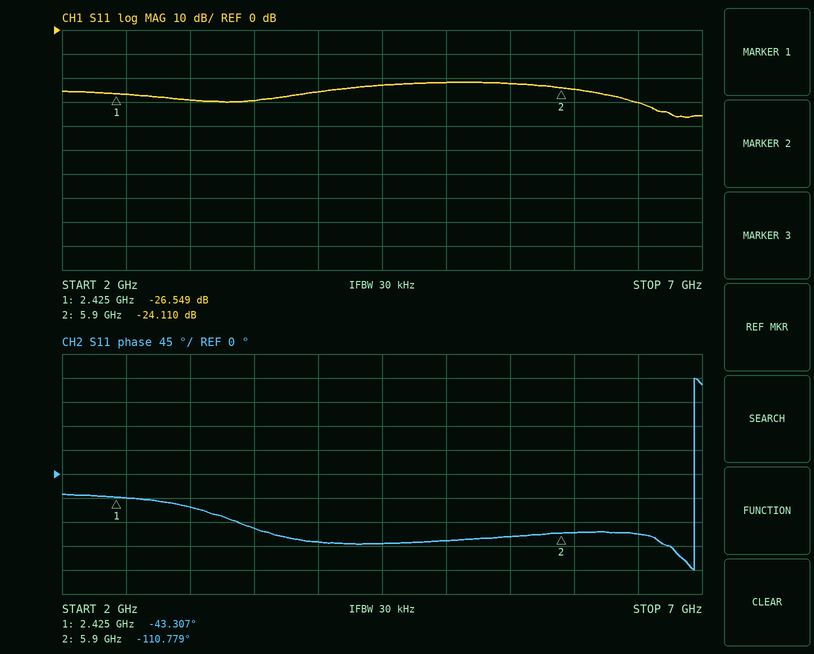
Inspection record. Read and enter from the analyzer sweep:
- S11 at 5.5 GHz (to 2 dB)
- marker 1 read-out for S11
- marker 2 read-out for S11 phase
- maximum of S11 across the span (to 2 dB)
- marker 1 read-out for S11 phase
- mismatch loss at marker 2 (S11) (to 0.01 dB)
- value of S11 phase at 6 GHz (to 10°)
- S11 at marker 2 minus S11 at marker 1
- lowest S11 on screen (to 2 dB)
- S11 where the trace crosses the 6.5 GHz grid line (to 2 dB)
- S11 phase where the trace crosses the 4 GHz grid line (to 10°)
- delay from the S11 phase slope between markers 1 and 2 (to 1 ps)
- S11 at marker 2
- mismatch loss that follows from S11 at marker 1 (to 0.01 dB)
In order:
-22 dB
-26.549 dB
-110.779°
-22 dB
-43.307°
0.02 dB
-110°
2.439 dB
-36 dB
-30 dB
-130°
54 ps
-24.110 dB
0.01 dB
